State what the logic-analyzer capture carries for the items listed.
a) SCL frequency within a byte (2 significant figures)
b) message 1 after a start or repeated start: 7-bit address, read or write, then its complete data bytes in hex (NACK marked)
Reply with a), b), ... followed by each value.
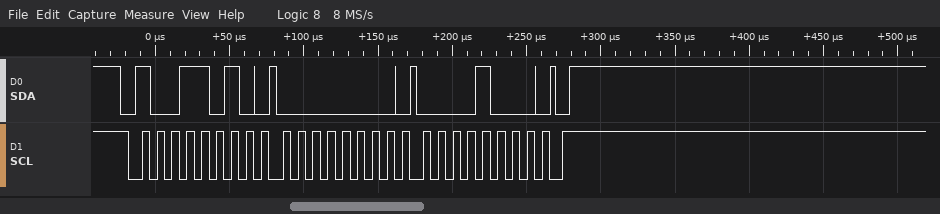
a) 100 kHz
b) 0x4D write: 00 08
